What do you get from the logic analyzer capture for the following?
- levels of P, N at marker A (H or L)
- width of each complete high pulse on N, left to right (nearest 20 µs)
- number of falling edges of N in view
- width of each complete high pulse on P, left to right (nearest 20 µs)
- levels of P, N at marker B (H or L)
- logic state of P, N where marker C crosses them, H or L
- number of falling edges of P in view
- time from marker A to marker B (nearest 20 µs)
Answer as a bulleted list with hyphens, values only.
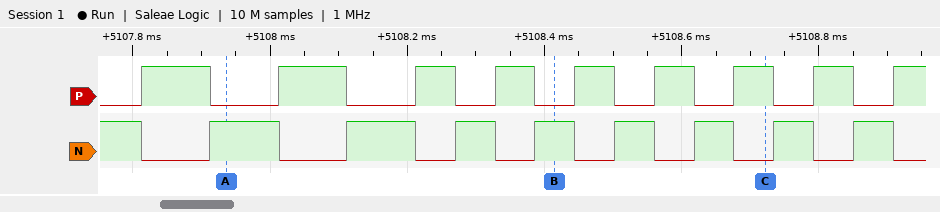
- P=L, N=H
- 100 µs, 100 µs, 60 µs, 60 µs, 60 µs, 60 µs, 60 µs, 60 µs
- 9
- 100 µs, 100 µs, 60 µs, 60 µs, 60 µs, 60 µs, 60 µs, 60 µs
- P=L, N=H
- P=H, N=L
- 8
- 480 µs
